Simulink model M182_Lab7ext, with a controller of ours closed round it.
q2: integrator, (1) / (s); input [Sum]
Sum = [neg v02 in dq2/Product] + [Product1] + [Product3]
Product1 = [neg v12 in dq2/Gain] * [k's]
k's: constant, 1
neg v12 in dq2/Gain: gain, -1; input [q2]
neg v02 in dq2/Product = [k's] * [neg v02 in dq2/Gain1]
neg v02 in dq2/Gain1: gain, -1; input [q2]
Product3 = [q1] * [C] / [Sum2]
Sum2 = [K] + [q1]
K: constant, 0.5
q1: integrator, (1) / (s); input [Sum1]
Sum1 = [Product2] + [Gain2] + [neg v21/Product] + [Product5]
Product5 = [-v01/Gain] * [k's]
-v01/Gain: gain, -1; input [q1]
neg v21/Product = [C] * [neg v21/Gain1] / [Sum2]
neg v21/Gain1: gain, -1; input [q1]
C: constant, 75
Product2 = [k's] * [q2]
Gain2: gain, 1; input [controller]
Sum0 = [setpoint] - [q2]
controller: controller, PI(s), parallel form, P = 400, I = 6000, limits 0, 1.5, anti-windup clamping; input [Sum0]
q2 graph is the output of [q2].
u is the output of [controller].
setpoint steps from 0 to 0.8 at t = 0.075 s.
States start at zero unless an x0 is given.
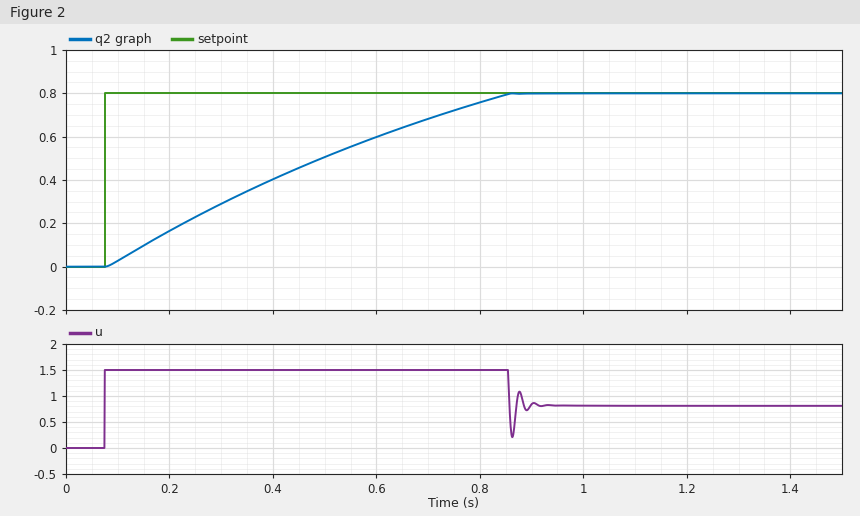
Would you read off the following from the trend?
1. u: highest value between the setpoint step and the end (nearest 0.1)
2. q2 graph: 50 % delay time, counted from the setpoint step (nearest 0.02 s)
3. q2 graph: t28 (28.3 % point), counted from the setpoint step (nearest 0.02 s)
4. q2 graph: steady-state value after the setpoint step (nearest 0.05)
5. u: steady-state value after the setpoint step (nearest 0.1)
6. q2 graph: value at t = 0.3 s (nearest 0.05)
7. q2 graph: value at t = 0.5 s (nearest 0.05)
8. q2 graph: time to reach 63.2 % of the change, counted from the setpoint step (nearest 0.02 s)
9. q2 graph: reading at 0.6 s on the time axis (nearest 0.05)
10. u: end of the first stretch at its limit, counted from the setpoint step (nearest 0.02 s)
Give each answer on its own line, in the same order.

1.5
0.32 s
0.18 s
0.80
0.8
0.30
0.50
0.42 s
0.60
0.78 s
